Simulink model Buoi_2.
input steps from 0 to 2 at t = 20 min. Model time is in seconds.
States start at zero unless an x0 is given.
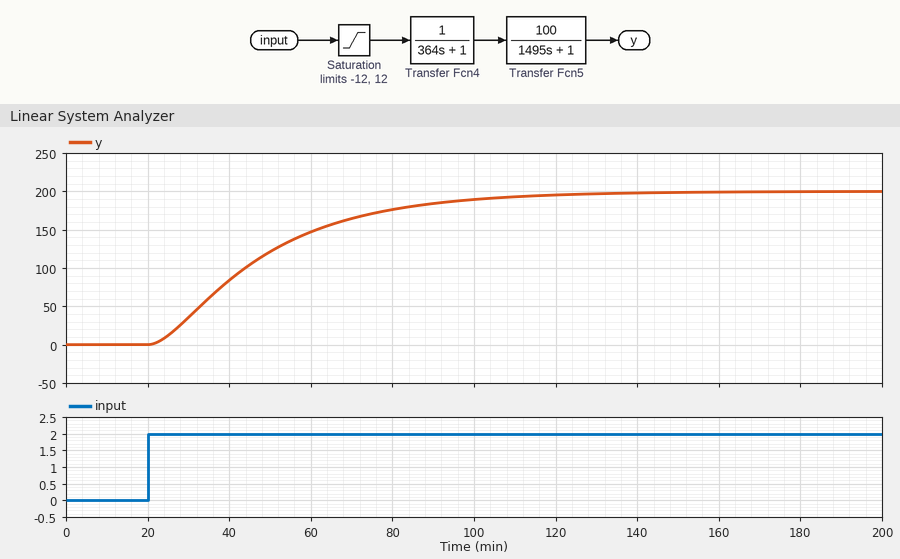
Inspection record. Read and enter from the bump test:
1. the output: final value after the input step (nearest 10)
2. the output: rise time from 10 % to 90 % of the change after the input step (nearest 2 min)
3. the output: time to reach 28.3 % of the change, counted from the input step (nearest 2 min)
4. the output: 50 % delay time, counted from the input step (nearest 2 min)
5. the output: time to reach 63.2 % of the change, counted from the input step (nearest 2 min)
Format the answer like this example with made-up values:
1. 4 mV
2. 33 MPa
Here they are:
1. 200
2. 58 min
3. 14 min
4. 24 min
5. 32 min
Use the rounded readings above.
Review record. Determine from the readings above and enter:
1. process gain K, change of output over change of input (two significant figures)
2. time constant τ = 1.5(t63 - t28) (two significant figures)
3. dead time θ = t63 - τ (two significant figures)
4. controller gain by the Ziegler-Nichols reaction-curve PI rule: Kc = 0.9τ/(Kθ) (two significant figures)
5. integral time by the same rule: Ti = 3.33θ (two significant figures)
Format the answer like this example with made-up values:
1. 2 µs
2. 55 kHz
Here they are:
1. 100
2. 27 min
3. 5.0 min
4. 0.049
5. 17 min
